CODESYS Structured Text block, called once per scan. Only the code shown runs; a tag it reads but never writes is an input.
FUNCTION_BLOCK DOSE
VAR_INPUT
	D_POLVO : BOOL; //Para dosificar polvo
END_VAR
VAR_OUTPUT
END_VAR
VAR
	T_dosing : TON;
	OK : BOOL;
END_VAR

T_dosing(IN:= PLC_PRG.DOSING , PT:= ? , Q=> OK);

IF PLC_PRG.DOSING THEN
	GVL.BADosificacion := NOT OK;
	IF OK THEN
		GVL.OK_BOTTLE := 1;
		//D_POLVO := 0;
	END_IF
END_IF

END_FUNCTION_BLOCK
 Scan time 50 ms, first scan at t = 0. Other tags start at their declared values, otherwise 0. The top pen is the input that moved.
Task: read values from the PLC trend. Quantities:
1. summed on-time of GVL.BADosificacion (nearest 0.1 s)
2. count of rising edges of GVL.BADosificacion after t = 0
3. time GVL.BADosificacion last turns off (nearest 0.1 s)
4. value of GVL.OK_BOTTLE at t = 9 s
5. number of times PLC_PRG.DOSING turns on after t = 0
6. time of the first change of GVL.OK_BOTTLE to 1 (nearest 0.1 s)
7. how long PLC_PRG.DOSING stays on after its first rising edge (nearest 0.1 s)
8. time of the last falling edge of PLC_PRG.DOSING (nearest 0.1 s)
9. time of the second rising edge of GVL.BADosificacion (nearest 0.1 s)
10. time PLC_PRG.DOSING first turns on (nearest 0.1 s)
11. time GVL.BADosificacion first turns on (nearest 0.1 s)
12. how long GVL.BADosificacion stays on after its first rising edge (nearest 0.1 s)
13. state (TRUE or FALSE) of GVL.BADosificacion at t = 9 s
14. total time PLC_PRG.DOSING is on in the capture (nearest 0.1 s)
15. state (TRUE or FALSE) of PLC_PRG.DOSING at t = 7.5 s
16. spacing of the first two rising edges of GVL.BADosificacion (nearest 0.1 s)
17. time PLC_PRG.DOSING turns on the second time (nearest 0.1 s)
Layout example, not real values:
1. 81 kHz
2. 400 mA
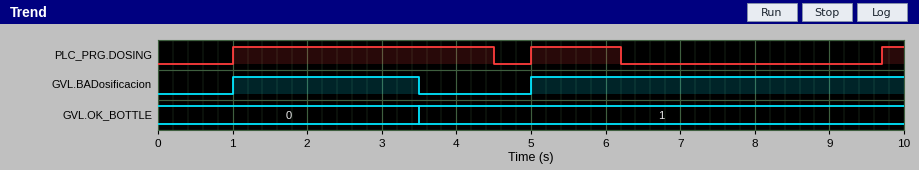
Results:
1. 7.5 s
2. 2
3. 3.5 s
4. 1
5. 3
6. 3.5 s
7. 3.5 s
8. 6.2 s
9. 5.0 s
10. 1.0 s
11. 1.0 s
12. 2.5 s
13. TRUE
14. 5.0 s
15. FALSE
16. 4.0 s
17. 5.0 s
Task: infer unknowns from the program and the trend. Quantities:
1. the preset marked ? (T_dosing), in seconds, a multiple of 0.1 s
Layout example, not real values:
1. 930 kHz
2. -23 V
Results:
1. 2.5 s
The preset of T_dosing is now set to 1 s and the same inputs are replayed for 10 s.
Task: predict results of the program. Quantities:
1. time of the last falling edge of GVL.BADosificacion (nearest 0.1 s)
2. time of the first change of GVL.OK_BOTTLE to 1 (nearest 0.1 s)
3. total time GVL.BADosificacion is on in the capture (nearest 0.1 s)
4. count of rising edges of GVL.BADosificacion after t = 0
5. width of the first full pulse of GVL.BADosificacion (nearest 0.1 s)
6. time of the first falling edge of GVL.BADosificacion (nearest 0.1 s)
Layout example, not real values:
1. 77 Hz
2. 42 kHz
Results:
1. 6.0 s
2. 2.0 s
3. 2.3 s
4. 3
5. 1.0 s
6. 2.0 s
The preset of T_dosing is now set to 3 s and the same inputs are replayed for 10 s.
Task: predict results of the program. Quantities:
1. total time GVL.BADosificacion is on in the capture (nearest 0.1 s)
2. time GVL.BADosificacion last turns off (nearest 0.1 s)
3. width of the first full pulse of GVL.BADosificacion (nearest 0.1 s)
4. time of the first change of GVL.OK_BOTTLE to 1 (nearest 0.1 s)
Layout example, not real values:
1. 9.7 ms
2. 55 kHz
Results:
1. 8.0 s
2. 4.0 s
3. 3.0 s
4. 4.0 s
